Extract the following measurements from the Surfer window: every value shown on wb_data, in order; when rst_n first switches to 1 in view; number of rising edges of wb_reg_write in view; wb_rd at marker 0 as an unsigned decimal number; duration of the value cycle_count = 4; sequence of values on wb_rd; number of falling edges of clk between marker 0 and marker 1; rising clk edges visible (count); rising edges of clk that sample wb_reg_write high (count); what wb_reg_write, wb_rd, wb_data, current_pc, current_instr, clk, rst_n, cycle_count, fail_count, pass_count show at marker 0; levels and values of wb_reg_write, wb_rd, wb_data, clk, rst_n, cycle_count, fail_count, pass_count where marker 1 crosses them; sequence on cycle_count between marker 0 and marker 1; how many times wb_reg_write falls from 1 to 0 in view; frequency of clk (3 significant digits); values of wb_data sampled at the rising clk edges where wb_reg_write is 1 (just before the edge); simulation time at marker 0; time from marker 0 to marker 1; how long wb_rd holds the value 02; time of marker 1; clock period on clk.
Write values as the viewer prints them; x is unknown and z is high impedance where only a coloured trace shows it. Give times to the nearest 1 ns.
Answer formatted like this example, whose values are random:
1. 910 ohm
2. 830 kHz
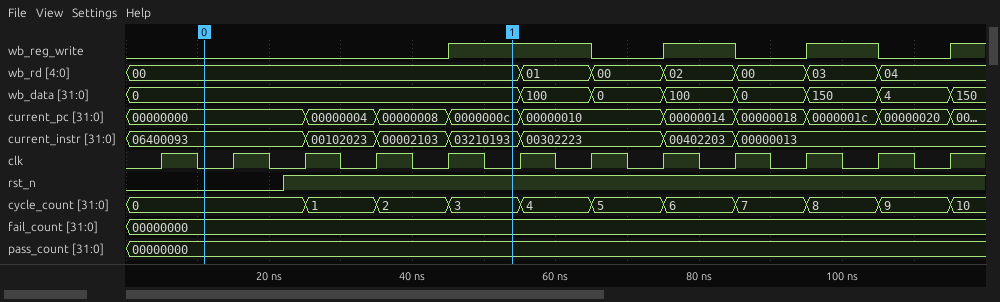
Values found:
1. 0, 100, 0, 100, 0, 150, 4, 150
2. 22 ns
3. 4
4. 0
5. 10 ns
6. 00, 01, 00, 02, 00, 03, 04
7. 4
8. 12
9. 4
10. wb_reg_write=0, wb_rd=00, wb_data=0, current_pc=00000000, current_instr=06400093, clk=0, rst_n=0, cycle_count=0, fail_count=00000000, pass_count=00000000
11. wb_reg_write=1, wb_rd=00, wb_data=0, clk=0, rst_n=1, cycle_count=3, fail_count=00000000, pass_count=00000000
12. 0, 1, 2, 3
13. 3
14. 100 MHz
15. 0, 100, 100, 150
16. 11 ns
17. 43 ns
18. 10 ns
19. 54 ns
20. 10 ns
